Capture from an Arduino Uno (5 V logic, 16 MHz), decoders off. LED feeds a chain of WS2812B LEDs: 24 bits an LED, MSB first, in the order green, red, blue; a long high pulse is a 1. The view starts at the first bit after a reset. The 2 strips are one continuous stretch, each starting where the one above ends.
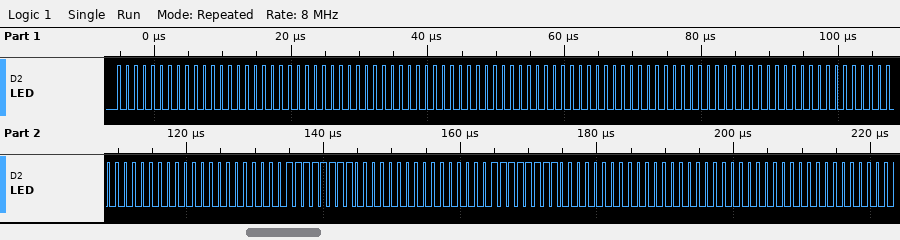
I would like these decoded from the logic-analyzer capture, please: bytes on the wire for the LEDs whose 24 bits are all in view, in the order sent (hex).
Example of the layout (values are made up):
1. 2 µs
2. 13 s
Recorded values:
1. 00 00 00 00 00 00 00 00 00 00 00 00 00 00 FF 00 00 FF 00 00 00
